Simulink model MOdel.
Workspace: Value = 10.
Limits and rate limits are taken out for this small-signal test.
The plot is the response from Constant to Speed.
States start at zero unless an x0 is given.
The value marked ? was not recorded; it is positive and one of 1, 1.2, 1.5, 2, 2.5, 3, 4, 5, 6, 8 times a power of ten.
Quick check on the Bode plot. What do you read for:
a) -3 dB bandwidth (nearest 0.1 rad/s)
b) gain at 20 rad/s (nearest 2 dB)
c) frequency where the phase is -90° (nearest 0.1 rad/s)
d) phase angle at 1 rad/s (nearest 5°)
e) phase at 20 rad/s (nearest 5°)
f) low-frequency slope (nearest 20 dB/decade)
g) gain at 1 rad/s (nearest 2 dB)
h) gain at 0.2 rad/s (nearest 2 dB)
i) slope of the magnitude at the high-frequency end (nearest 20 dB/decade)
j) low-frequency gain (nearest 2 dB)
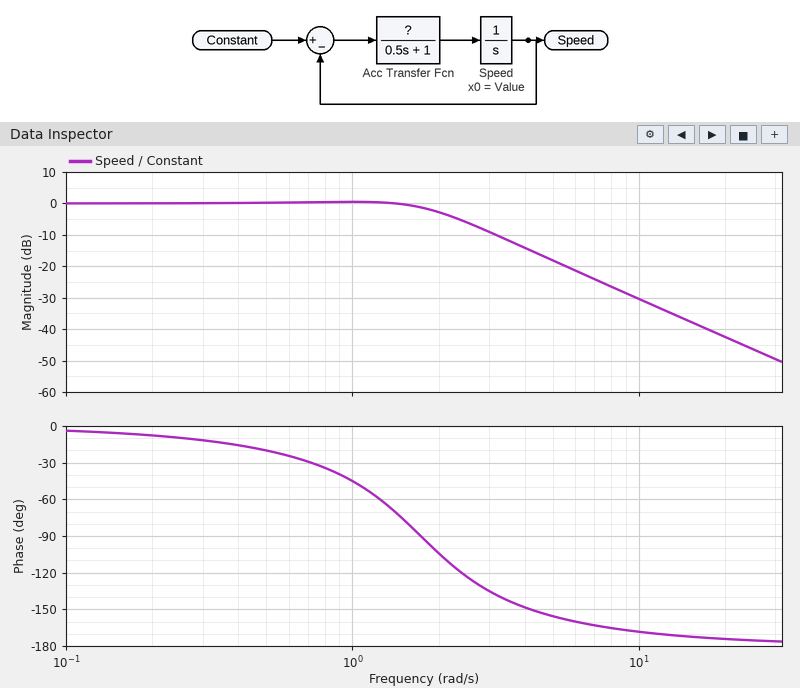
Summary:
2.0 rad/s
-42 dB
1.7 rad/s
-45°
-175°
0 dB/decade
0 dB
0 dB
-40 dB/decade
0 dB
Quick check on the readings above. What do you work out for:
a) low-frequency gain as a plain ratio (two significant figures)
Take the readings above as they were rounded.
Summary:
1.0
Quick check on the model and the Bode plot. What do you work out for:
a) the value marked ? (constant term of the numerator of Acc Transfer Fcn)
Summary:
1.5
